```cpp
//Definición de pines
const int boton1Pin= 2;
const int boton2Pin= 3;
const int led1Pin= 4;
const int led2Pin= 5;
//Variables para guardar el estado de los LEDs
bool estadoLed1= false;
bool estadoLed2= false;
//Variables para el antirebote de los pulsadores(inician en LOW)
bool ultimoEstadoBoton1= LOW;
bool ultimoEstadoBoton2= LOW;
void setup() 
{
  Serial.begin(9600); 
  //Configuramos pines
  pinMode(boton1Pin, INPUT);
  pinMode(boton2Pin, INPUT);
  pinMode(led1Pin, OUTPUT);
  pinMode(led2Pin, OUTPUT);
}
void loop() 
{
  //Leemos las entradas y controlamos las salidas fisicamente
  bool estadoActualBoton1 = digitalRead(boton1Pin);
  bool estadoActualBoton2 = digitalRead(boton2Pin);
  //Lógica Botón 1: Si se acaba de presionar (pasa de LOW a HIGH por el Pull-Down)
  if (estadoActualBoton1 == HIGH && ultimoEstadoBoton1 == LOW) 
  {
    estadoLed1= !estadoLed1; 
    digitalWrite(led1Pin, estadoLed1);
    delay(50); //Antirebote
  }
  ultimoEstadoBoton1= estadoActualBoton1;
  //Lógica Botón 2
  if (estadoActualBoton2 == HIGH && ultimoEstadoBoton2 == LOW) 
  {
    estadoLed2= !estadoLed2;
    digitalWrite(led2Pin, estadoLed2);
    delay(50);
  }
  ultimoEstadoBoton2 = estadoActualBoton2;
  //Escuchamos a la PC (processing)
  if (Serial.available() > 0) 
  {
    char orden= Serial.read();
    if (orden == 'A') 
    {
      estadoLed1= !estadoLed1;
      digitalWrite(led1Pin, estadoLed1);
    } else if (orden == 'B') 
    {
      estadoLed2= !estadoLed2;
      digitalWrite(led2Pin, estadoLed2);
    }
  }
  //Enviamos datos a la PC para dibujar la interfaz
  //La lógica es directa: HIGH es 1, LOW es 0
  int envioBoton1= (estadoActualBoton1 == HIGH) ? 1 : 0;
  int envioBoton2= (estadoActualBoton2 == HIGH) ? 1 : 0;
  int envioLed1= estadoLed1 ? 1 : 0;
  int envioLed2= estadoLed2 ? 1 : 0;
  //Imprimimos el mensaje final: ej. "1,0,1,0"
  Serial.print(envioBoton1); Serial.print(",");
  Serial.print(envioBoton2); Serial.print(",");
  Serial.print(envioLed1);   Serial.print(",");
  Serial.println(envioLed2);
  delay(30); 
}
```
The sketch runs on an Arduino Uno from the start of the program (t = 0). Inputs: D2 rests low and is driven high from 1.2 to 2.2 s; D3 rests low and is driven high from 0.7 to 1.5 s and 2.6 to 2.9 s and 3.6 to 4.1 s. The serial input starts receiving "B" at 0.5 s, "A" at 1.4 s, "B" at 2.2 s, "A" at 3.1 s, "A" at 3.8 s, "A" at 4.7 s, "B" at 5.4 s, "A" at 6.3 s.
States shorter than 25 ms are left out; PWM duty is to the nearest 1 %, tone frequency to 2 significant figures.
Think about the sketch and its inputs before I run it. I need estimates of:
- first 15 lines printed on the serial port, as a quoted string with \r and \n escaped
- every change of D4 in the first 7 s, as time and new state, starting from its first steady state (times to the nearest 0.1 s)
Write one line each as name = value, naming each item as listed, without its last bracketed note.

first 15 lines printed on the serial port, as a quoted string with \r and \n escaped = "0,0,0,0\r\n0,0,0,0\r\n0,0,0,0\r\n0,0,0,0\r\n0,0,0,0\r\n0,0,0,0\r\n0,0,0,0\r\n0,0,0,0\r\n0,0,0,0\r\n0,0,0,0\r\n0,0,0,0\r\n0,0,0,0\r\n0,0,0,0\r\n0,0,0,0\r\n0,0,0,0\r\n"
every change of D4 in the first 7 s, as time and new state, starting from its first steady state = 0 s low; 1.2 s high; 1.4 s low; 3.1 s high; 3.8 s low; 4.7 s high; 6.3 s low
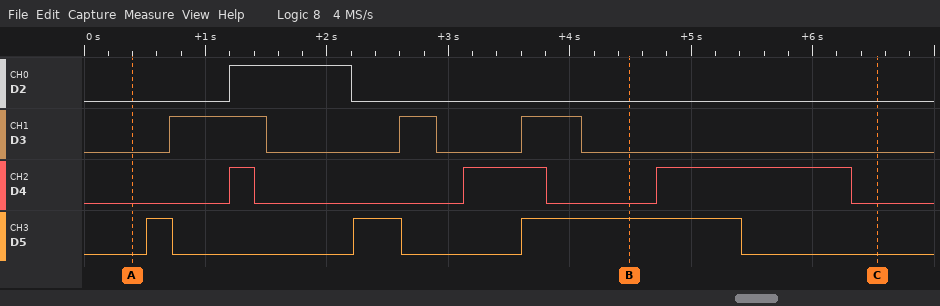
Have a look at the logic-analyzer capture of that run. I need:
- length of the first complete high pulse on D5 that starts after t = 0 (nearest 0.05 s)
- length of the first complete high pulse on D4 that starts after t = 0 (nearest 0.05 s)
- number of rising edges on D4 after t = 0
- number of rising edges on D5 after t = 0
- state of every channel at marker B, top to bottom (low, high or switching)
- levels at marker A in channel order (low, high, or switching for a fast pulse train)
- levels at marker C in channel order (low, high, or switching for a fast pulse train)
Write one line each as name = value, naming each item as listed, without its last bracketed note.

length of the first complete high pulse on D5 that starts after t = 0 = 0.20 s
length of the first complete high pulse on D4 that starts after t = 0 = 0.20 s
number of rising edges on D4 after t = 0 = 3
number of rising edges on D5 after t = 0 = 3
state of every channel at marker B, top to bottom = D2 low, D3 low, D4 low, D5 high
levels at marker A in channel order = D2 low, D3 low, D4 low, D5 low
levels at marker C in channel order = D2 low, D3 low, D4 low, D5 low
